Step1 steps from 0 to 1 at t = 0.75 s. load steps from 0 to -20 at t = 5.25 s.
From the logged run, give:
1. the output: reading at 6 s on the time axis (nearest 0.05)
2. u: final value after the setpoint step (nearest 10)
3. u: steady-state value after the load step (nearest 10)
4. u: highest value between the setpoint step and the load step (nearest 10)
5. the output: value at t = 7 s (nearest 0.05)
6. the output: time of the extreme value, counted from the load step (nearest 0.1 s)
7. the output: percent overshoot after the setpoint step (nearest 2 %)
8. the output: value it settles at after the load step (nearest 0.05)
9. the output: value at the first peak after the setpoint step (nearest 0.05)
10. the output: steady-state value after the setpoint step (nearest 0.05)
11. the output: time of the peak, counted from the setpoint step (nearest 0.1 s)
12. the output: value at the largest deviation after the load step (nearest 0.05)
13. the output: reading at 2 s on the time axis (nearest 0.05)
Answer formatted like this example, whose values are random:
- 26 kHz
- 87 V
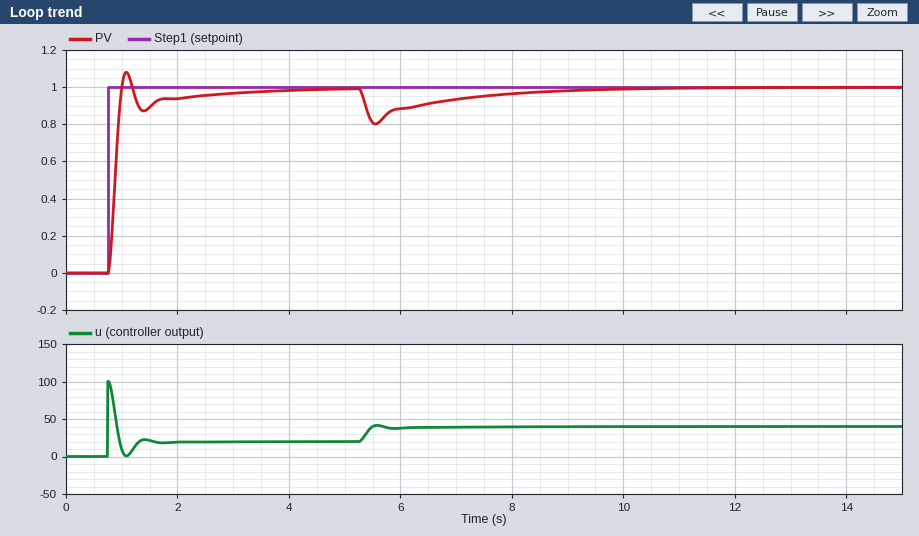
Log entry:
- 0.90
- 20
- 40
- 100
- 0.95
- 0.3 s
- 8 %
- 1.00
- 1.10
- 1.00
- 0.3 s
- 0.80
- 0.95
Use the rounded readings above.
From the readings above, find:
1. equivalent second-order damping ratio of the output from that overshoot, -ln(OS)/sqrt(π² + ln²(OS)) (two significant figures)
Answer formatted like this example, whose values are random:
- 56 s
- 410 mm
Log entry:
- 0.63
